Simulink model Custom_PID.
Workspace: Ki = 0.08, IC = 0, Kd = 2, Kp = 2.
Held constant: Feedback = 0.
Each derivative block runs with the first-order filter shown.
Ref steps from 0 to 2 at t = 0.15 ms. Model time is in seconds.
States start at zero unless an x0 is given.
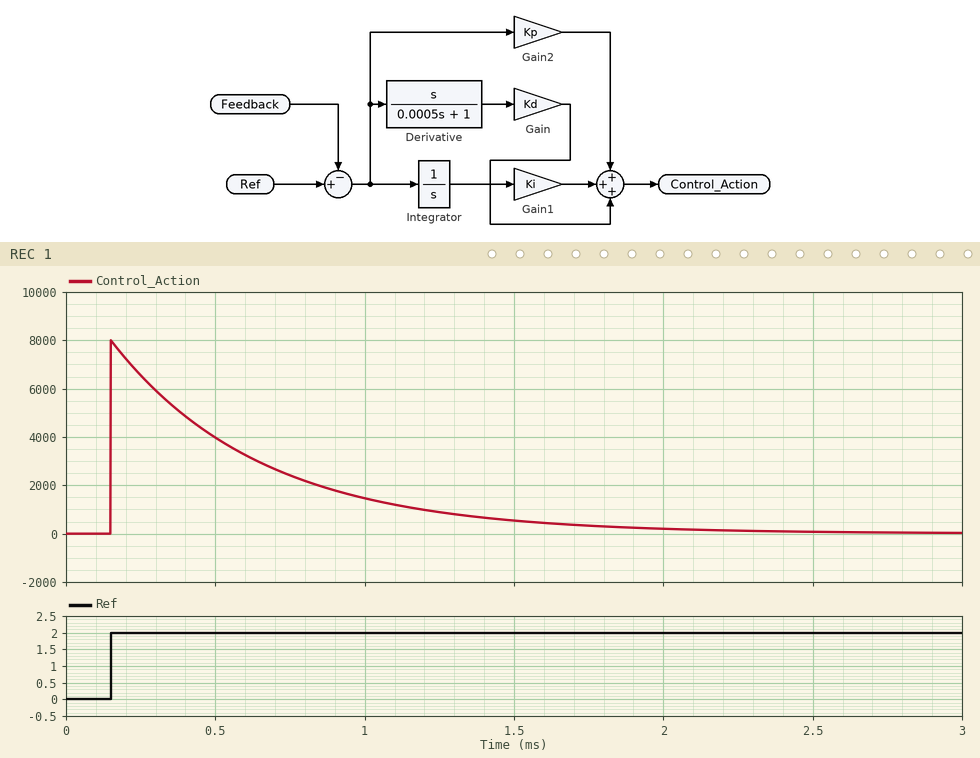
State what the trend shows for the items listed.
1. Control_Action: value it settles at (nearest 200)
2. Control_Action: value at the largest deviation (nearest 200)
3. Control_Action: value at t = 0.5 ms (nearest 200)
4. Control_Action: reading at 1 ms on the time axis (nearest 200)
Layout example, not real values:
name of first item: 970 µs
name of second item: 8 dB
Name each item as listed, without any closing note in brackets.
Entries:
Control_Action: value it settles at: 0
Control_Action: value at the largest deviation: 8000
Control_Action: value at t = 0.5 ms: 4000
Control_Action: reading at 1 ms on the time axis: 1400
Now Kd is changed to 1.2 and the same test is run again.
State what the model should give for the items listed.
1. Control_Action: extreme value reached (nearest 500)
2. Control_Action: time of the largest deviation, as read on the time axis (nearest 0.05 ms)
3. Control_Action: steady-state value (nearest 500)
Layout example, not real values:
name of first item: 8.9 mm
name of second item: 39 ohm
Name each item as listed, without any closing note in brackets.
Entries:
Control_Action: extreme value reached: 5000
Control_Action: time of the largest deviation, as read on the time axis: 0.15 ms
Control_Action: steady-state value: 0
